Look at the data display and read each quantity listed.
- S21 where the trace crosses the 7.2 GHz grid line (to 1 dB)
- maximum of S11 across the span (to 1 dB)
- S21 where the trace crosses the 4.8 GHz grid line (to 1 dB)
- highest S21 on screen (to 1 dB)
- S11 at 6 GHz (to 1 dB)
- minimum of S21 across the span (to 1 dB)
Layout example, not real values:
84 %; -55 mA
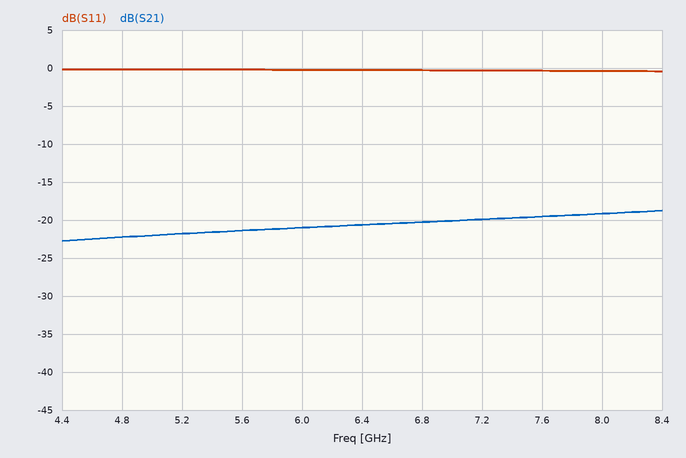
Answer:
-20 dB; 0 dB; -22 dB; -19 dB; 0 dB; -23 dB
